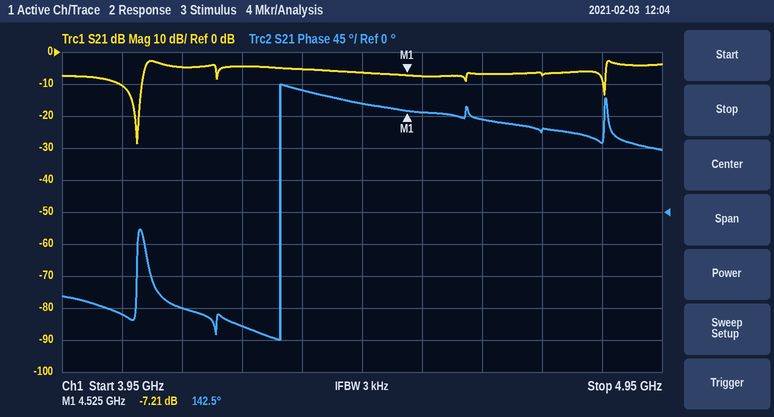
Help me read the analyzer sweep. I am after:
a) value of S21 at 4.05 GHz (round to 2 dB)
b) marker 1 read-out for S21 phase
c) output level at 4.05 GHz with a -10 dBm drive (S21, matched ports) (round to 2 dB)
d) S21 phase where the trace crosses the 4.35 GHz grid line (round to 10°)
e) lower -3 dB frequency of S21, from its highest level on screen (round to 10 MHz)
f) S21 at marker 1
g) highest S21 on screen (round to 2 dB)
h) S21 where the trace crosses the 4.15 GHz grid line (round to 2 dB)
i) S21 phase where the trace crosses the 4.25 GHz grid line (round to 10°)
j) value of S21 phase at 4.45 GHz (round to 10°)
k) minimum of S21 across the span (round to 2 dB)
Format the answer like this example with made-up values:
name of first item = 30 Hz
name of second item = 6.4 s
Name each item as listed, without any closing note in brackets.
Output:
value of S21 at 4.05 GHz = -10 dB
marker 1 read-out for S21 phase = 142.5°
output level at 4.05 GHz with a -10 dBm drive (S21, matched ports) = -20 dBm
S21 phase where the trace crosses the 4.35 GHz grid line = 170°
lower -3 dB frequency of S21, from its highest level on screen = 4.09 GHz
S21 at marker 1 = -7.21 dB
highest S21 on screen = -2 dB
S21 where the trace crosses the 4.15 GHz grid line = -4 dB
S21 phase where the trace crosses the 4.25 GHz grid line = -160°
value of S21 phase at 4.45 GHz = 150°
minimum of S21 across the span = -28 dB
